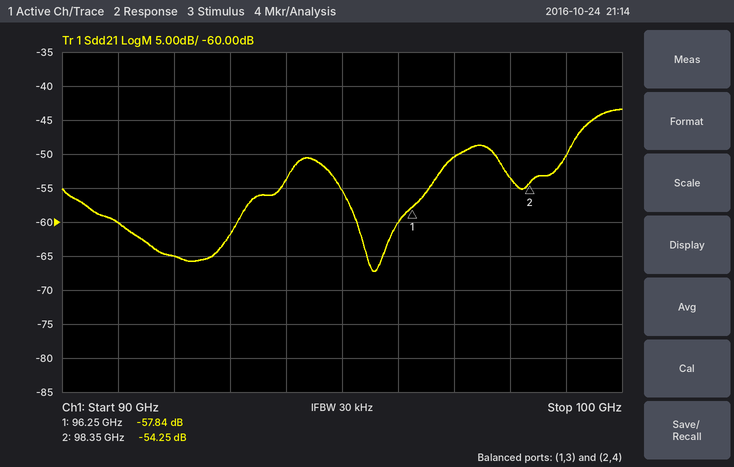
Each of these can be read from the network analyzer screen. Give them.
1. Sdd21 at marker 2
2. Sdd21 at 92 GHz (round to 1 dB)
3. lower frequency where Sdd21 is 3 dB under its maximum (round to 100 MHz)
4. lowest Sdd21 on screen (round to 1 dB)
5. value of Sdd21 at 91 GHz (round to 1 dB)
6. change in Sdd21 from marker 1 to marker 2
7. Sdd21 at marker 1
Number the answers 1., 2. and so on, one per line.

1. -54.25 dB
2. -65 dB
3. 99.3 GHz
4. -67 dB
5. -60 dB
6. 3.59 dB
7. -57.84 dB
